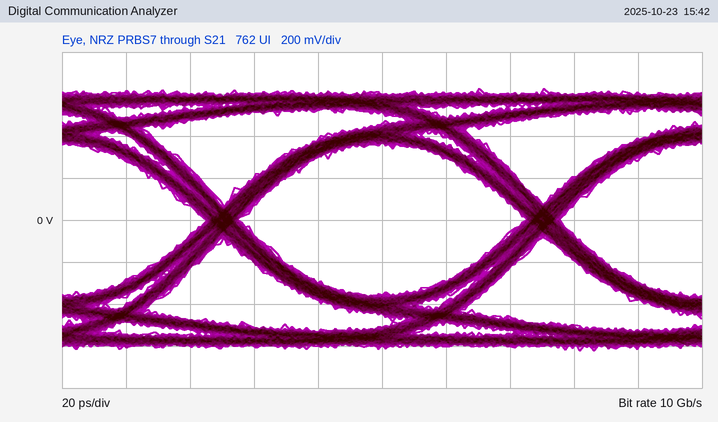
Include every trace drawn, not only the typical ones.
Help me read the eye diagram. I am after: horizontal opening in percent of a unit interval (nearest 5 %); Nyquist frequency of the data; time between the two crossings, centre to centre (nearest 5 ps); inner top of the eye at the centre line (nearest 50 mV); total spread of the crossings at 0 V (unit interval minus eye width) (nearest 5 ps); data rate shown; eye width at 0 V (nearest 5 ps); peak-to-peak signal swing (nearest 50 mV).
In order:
90 %
5 GHz
100 ps
350 mV
10 ps
10 Gb/s
90 ps
1.25 V
